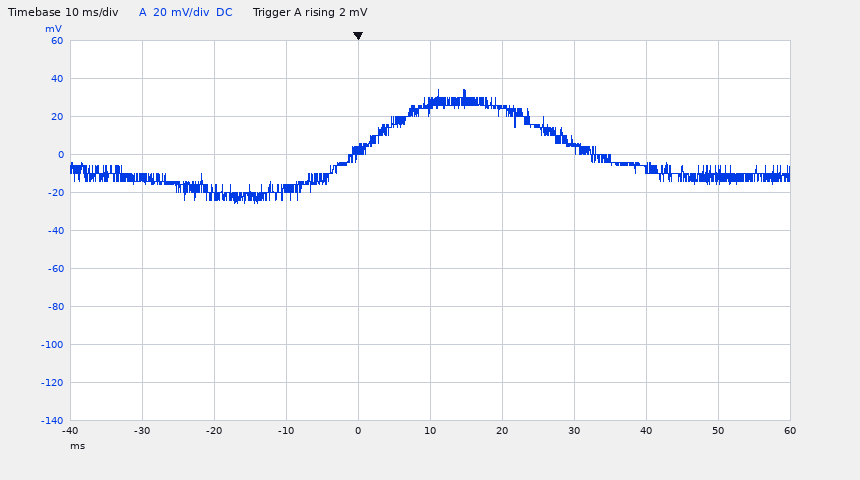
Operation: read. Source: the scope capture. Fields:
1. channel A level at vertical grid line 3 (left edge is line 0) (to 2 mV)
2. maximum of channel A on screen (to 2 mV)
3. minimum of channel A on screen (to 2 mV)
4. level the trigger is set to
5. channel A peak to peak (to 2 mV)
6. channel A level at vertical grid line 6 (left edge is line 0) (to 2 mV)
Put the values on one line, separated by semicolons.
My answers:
-18 mV; 34 mV; -26 mV; 2 mV; 60 mV; 24 mV
